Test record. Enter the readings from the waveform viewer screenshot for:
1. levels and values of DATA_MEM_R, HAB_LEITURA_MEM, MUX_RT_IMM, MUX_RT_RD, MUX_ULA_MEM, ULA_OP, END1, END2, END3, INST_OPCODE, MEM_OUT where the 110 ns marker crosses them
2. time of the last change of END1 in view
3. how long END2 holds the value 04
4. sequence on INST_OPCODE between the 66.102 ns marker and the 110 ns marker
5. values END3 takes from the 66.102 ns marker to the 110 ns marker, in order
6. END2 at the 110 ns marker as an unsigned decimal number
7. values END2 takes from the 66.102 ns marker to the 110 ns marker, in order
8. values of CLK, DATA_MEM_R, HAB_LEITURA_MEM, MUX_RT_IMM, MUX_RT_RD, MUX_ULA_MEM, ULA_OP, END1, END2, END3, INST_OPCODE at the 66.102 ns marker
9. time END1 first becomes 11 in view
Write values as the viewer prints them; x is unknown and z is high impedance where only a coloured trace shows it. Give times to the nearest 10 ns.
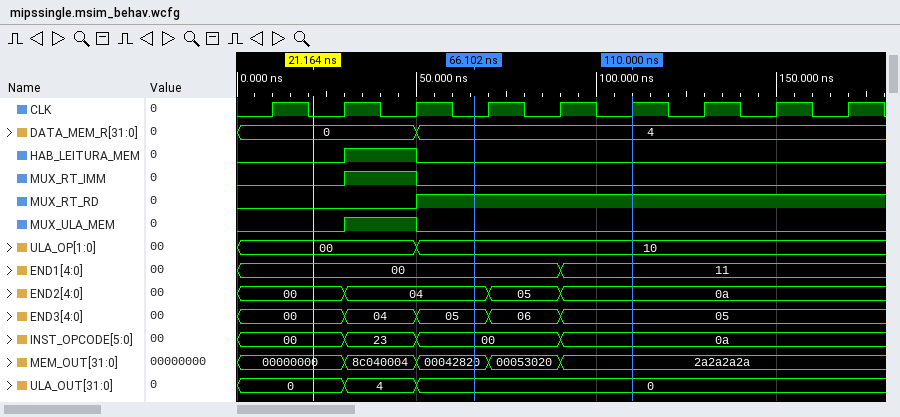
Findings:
DATA_MEM_R=4, HAB_LEITURA_MEM=0, MUX_RT_IMM=0, MUX_RT_RD=1, MUX_ULA_MEM=0, ULA_OP=10, END1=11, END2=0a, END3=05, INST_OPCODE=0a, MEM_OUT=2a2a2a2a
90 ns
40 ns
00, 0a
05, 06, 05
10
04, 05, 0a
CLK=0, DATA_MEM_R=4, HAB_LEITURA_MEM=0, MUX_RT_IMM=0, MUX_RT_RD=1, MUX_ULA_MEM=0, ULA_OP=10, END1=00, END2=04, END3=05, INST_OPCODE=00
90 ns
